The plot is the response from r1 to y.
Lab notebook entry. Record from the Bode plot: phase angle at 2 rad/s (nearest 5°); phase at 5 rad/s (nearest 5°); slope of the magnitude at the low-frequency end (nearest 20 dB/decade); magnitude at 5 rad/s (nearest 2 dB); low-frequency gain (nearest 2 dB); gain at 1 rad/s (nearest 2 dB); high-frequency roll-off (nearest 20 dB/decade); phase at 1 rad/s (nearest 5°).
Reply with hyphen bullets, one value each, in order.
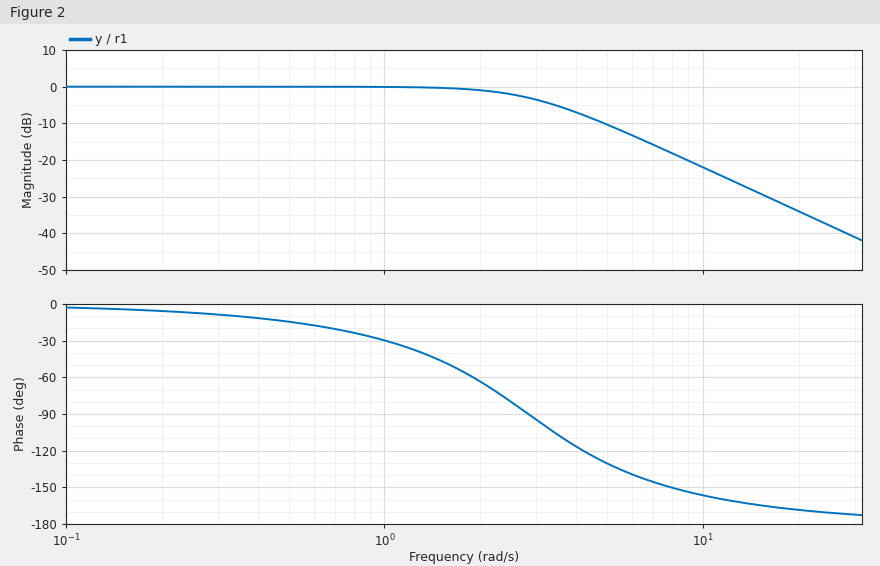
- -65°
- -130°
- 0 dB/decade
- -10 dB
- 0 dB
- 0 dB
- -40 dB/decade
- -30°
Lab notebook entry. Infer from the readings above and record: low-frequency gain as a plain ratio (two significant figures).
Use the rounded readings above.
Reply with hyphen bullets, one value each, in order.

- 1.0
